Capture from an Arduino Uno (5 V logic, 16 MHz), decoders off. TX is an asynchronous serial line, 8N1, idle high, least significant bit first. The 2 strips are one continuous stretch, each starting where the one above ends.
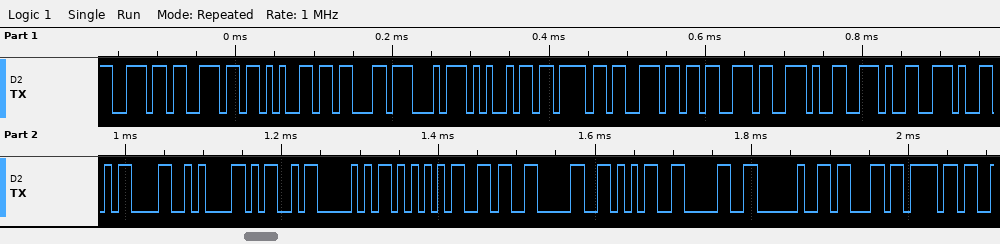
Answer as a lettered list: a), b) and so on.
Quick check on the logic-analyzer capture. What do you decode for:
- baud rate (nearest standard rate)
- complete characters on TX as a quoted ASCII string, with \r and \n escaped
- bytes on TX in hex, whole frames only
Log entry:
a) 115200 baud
b) "nnections...\r\nMPU6050 co"
c) 6E 6E 65 63 74 69 6F 6E 73 2E 2E 2E 0D 0A 4D 50 55 36 30 35 30 20 63 6F
